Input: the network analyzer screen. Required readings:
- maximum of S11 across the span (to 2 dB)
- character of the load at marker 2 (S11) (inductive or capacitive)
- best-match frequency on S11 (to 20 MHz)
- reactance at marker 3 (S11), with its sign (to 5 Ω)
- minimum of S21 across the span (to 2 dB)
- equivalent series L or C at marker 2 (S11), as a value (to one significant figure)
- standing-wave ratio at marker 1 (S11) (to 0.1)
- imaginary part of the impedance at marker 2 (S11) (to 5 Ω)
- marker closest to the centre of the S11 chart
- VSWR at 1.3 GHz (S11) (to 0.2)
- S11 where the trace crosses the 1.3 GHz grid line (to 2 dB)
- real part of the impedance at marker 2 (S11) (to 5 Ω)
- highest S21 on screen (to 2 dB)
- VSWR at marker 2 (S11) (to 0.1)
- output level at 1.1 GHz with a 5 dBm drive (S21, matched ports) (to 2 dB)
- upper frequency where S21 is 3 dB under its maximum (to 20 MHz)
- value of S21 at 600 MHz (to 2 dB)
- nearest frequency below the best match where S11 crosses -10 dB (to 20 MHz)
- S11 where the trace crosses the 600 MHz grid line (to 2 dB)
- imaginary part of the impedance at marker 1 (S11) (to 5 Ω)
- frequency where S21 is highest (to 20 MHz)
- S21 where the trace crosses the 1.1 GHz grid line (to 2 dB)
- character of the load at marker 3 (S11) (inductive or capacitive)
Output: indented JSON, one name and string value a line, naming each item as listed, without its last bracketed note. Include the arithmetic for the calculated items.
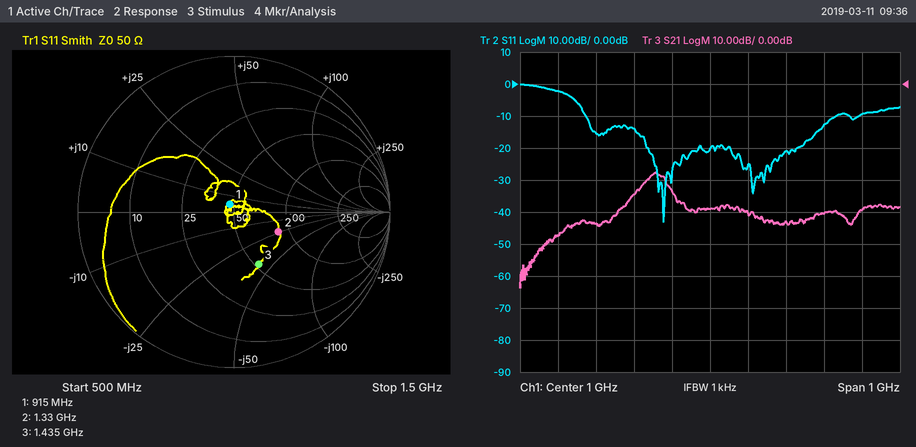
{
  "maximum of S11 across the span": "0 dB",
  "character of the load at marker 2 (S11)": "capacitive",
  "best-match frequency on S11": "880 MHz",
  "reactance at marker 3 (S11), with its sign": "-40 Ω",
  "minimum of S21 across the span": "-64 dB",
  "equivalent series L or C at marker 2 (S11), as a value": "C = 1/(2π × 1.33 GHz × 25 Ω) ≈ 5 pF",
  "standing-wave ratio at marker 1 (S11)": "1.1",
  "imaginary part of the impedance at marker 2 (S11)": "-25 Ω",
  "marker closest to the centre of the S11 chart": "marker 1",
  "VSWR at 1.3 GHz (S11)": "|Γ| = 10^(-12/20) = 0.2512; VSWR = (1 + 0.2512)/(1 − 0.2512) ≈ 1.67, so 1.6 to the nearest 0.2",
  "S11 where the trace crosses the 1.3 GHz grid line": "-12 dB",
  "real part of the impedance at marker 2 (S11)": "85 Ω",
  "highest S21 on screen": "-28 dB",
  "VSWR at marker 2 (S11)": "1.9",
  "output level at 1.1 GHz with a 5 dBm drive (S21, matched ports)": "5 dBm + (-40 dB) = -36 dBm",
  "upper frequency where S21 is 3 dB under its maximum": "880 MHz",
  "value of S21 at 600 MHz": "-48 dB",
  "nearest frequency below the best match where S11 crosses -10 dB": "680 MHz",
  "S11 where the trace crosses the 600 MHz grid line": "-2 dB",
  "imaginary part of the impedance at marker 1 (S11)": "+5 Ω",
  "frequency where S21 is highest": "860 MHz",
  "S21 where the trace crosses the 1.1 GHz grid line": "-40 dB",
  "character of the load at marker 3 (S11)": "capacitive"
}
